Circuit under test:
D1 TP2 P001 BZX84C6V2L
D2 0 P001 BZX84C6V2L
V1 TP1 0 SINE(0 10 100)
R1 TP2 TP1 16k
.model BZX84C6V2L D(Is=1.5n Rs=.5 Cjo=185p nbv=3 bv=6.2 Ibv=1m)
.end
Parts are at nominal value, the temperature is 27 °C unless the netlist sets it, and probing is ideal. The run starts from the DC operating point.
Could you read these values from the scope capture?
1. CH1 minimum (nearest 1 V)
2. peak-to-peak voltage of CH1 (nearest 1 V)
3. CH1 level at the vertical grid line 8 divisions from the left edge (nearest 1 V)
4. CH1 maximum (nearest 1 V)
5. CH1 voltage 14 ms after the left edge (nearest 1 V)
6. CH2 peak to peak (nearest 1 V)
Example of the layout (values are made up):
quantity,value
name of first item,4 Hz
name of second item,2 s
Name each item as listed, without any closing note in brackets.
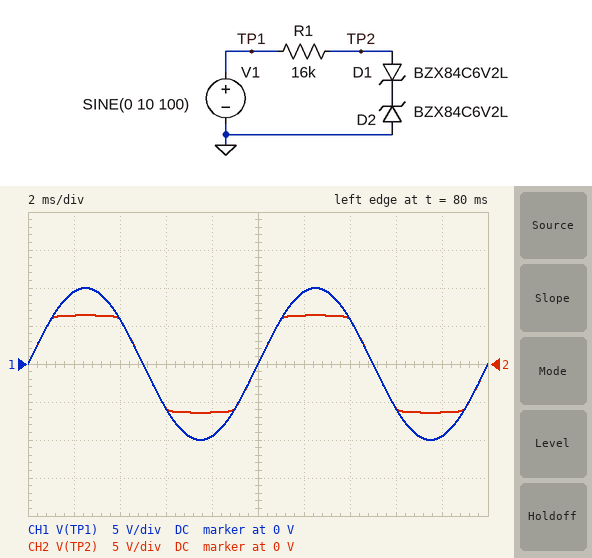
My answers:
quantity,value
CH1 minimum,-10 V
peak-to-peak voltage of CH1,20 V
CH1 level at the vertical grid line 8 divisions from the left edge,-6 V
CH1 maximum,10 V
CH1 voltage 14 ms after the left edge,6 V
CH2 peak to peak,13 V
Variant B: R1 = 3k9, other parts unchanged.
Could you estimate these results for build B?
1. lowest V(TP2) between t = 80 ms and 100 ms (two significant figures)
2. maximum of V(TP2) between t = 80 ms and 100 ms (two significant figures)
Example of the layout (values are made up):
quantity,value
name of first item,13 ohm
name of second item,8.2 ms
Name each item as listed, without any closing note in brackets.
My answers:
quantity,value
lowest V(TP2) between t = 80 ms and 100 ms,-6.5 V
maximum of V(TP2) between t = 80 ms and 100 ms,6.5 V
